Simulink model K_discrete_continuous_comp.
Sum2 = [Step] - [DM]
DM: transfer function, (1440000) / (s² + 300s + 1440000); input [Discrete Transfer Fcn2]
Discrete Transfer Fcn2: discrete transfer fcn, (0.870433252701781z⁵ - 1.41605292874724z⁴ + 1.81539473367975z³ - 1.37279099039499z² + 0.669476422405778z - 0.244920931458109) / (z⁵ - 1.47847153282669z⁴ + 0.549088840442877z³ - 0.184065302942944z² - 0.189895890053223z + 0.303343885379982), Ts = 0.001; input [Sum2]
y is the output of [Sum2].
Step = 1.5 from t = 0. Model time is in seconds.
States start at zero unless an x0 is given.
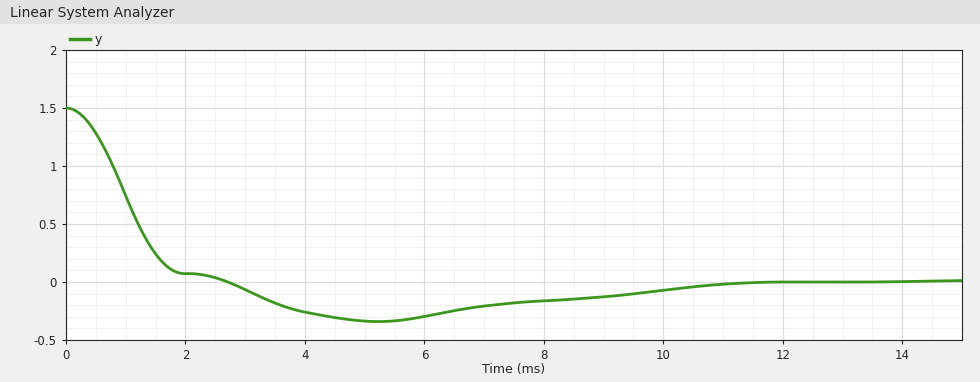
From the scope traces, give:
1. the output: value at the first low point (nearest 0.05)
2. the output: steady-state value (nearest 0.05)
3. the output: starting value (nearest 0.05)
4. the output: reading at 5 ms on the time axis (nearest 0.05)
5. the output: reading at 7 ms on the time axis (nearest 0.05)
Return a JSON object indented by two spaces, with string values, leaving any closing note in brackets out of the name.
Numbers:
{
  "the output: value at the first low point": "-0.35",
  "the output: steady-state value": "0.00",
  "the output: starting value": "1.50",
  "the output: reading at 5 ms on the time axis": "-0.35",
  "the output: reading at 7 ms on the time axis": "-0.20"
}
